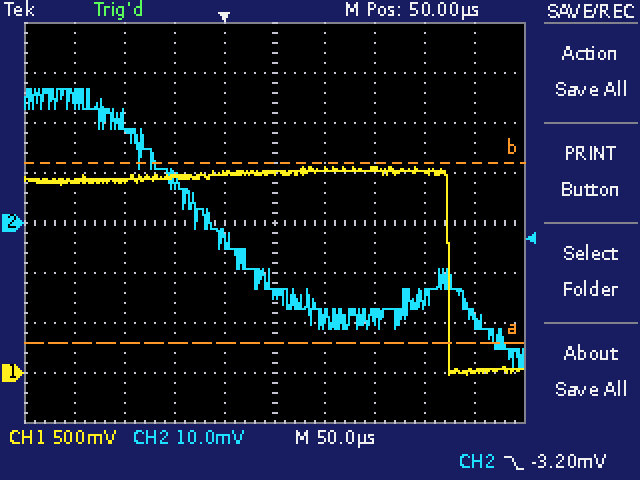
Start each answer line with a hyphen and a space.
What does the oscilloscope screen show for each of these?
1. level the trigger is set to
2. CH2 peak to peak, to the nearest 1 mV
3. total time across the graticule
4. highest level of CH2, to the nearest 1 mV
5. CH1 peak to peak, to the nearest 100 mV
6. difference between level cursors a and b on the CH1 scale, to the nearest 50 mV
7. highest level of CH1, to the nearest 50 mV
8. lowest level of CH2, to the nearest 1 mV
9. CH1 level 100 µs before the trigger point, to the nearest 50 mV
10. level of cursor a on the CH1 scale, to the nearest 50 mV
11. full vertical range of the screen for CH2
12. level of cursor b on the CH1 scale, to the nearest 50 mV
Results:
- -3.20 mV
- 56 mV
- 500 µs
- 27 mV
- 2.10 V
- 1.80 V
- 2.05 V
- -29 mV
- 1.90 V
- 300 mV
- 80 mV
- 2.10 V
